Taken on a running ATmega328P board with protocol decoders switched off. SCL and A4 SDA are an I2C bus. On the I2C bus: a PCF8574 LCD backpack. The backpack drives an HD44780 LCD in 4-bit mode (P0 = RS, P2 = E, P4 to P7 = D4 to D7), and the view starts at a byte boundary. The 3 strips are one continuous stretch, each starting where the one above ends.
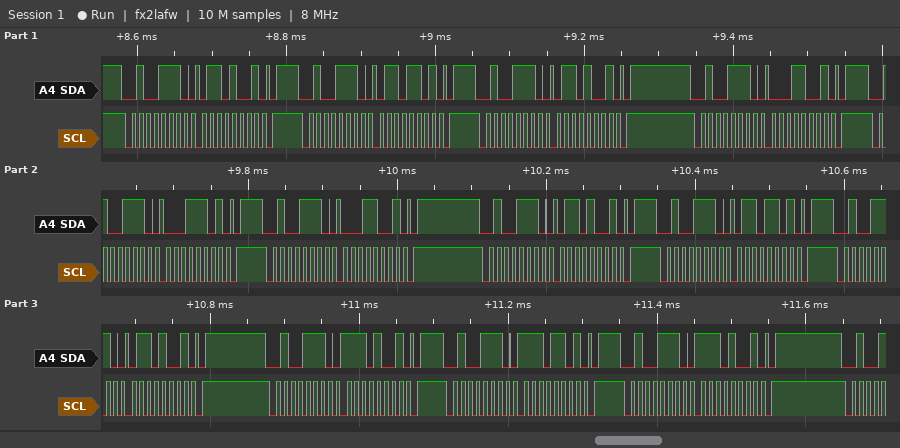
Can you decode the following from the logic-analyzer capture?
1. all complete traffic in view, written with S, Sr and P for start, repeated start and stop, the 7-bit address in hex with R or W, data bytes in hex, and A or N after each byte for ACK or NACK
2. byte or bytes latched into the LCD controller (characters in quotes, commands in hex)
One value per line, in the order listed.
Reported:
S 27W A 69 A P S 27W A 6D A P S 27W A 69 A P S 27W A 19 A P S 27W A 1D A P S 27W A 19 A P S 27W A 69 A P S 27W A 6D A P S 27W A 69 A P S 27W A E9 A P S 27W A ED A P S 27W A E9 A P
'a' 'n'
